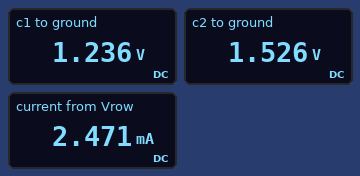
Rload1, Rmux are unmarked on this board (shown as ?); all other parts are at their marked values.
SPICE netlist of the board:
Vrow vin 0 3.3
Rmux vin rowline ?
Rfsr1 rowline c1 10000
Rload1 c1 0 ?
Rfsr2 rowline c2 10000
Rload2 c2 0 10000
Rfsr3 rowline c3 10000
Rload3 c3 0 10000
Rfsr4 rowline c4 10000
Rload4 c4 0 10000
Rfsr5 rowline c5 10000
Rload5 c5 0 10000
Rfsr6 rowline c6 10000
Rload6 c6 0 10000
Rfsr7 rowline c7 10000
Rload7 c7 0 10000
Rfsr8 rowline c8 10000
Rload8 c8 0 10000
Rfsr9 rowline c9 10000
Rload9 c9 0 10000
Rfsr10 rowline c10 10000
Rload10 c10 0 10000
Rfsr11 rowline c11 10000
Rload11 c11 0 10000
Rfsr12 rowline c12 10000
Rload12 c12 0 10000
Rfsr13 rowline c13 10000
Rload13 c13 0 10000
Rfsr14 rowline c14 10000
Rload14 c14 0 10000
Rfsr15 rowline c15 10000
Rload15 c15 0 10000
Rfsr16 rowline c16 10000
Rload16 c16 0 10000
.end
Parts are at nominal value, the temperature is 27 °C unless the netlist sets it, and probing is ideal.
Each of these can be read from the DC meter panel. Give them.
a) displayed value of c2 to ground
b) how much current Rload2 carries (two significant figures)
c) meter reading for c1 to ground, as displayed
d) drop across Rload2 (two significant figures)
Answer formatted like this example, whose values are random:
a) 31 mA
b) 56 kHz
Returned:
a) 1.526 V
b) 150 µA
c) 1.236 V
d) 1.5 V
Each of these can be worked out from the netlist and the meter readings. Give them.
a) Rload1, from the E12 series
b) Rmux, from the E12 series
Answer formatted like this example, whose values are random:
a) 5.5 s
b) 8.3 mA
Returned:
a) 6.8 kΩ
b) 100 Ω
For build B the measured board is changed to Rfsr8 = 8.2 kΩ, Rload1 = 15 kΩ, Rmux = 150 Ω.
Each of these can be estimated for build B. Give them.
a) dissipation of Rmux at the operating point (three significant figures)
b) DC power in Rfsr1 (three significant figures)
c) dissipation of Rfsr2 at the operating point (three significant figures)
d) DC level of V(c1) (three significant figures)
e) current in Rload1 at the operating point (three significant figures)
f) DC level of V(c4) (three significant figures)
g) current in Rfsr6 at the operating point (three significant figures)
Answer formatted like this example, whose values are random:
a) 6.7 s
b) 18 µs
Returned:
a) 824 µW
b) 139 µW
c) 217 µW
d) 1.77 V
e) 118 µA
f) 1.47 V
g) 147 µA
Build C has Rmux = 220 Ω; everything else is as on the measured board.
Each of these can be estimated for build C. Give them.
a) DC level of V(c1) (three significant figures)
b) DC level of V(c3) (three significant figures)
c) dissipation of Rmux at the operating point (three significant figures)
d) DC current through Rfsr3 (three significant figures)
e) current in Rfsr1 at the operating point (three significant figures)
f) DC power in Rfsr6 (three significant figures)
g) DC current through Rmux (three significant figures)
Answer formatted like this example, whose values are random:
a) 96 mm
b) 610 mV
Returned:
a) 1.13 V
b) 1.40 V
c) 1.13 mW
d) 140 µA
e) 167 µA
f) 196 µW
g) 2.27 mA
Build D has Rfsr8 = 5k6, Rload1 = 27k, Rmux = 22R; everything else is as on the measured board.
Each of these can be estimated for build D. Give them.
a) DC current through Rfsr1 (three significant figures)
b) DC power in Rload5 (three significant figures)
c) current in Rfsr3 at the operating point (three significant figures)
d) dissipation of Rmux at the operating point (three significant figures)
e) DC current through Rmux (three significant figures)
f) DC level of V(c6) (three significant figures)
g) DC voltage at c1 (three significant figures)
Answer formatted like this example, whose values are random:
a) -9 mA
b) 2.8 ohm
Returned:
a) 87.7 µA
b) 263 µW
c) 162 µA
d) 145 µW
e) 2.57 mA
f) 1.62 V
g) 2.37 V
